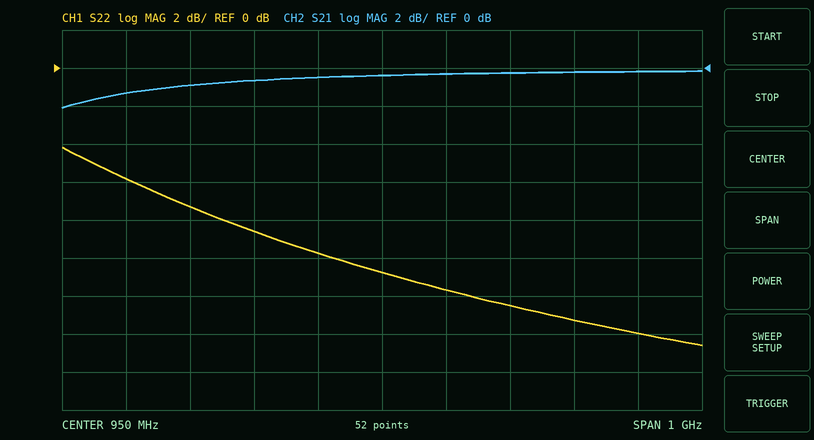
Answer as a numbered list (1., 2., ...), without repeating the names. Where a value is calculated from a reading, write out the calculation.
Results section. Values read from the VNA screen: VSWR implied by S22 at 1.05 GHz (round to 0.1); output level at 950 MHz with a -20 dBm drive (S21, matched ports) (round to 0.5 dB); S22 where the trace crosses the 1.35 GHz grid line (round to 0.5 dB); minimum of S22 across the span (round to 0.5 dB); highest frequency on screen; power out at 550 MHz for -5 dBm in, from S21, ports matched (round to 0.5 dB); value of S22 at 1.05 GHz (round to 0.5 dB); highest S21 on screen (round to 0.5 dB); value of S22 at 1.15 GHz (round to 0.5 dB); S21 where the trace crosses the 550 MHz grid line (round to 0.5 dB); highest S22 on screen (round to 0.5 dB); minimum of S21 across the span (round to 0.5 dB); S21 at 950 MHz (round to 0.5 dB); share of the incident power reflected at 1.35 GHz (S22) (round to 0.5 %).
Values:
1. |Γ| = 10^(-11.5/20) = 0.2661; VSWR = (1 + 0.2661)/(1 − 0.2661) ≈ 1.7
2. -20 dBm + (-0.5 dB) = -20.5 dBm
3. -14.0 dB
4. -14.5 dB
5. 1.45 GHz
6. -5 dBm + (-1.5 dB) = -6.5 dBm
7. -11.5 dB
8. 0.0 dB
9. -12.5 dB
10. -1.5 dB
11. -4.0 dB
12. -2.0 dB
13. -0.5 dB
14. 10^(-14/10) ≈ 4.0 %
